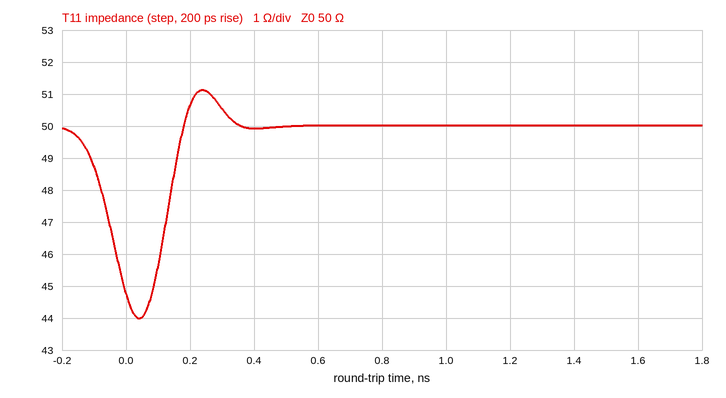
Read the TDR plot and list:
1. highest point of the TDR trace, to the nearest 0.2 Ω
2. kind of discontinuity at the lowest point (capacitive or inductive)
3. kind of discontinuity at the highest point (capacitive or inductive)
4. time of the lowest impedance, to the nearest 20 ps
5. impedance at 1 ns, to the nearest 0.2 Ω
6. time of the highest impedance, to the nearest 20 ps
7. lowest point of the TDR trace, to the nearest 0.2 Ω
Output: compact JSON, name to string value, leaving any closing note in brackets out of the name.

{"highest point of the TDR trace, to the nearest 0.2 Ω": "51.2 Ω", "kind of discontinuity at the lowest point": "capacitive", "kind of discontinuity at the highest point": "inductive", "time of the lowest impedance, to the nearest 20 ps": "40 ps", "impedance at 1 ns, to the nearest 0.2 Ω": "50.0 Ω", "time of the highest impedance, to the nearest 20 ps": "240 ps", "lowest point of the TDR trace, to the nearest 0.2 Ω": "44.0 Ω"}
